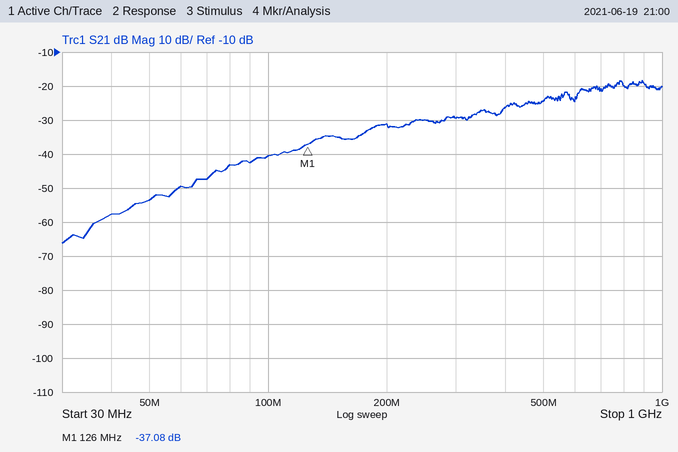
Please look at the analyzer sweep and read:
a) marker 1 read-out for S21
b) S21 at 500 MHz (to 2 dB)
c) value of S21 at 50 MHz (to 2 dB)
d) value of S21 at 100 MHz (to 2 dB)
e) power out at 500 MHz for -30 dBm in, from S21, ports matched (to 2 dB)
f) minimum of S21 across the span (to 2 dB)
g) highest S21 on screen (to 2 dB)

-37.08 dB
-24 dB
-54 dB
-40 dB
-54 dBm
-66 dB
-18 dB
